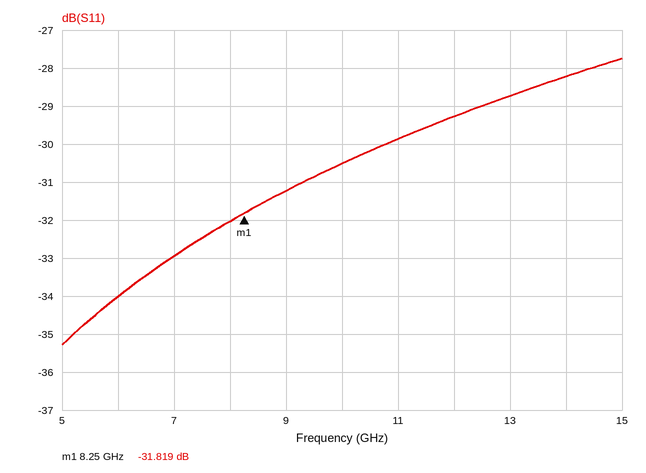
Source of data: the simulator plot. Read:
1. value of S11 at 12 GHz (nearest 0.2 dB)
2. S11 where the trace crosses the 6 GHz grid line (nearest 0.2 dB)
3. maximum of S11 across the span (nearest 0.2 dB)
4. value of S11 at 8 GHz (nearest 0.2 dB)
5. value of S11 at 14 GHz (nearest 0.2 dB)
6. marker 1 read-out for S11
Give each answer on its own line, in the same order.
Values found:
-29.2 dB
-34.0 dB
-27.8 dB
-32.0 dB
-28.2 dB
-31.819 dB
